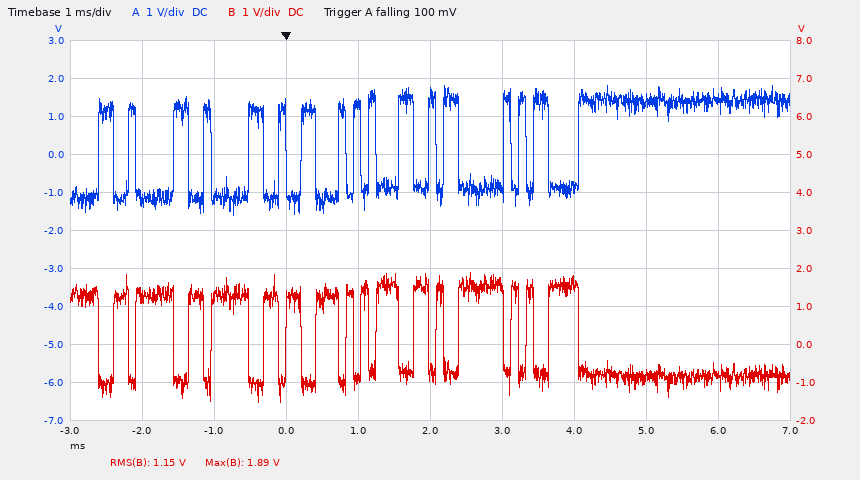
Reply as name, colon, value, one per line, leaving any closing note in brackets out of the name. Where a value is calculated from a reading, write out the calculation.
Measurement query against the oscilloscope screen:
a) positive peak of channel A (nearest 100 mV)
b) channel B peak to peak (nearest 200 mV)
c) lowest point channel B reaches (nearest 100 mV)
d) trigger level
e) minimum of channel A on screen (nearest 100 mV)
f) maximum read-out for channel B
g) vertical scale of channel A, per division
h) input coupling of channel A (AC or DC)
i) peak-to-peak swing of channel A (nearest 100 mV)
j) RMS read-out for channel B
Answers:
positive peak of channel A: 1.8 V
channel B peak to peak: 3.4 V
lowest point channel B reaches: -1.5 V
trigger level: 100 mV
minimum of channel A on screen: -1.6 V
maximum read-out for channel B: 1.89 V
vertical scale of channel A, per division: 1 V
input coupling of channel A: DC
peak-to-peak swing of channel A: 1.8 V − (-1.6 V) = 3.4 V
RMS read-out for channel B: 1.15 V
